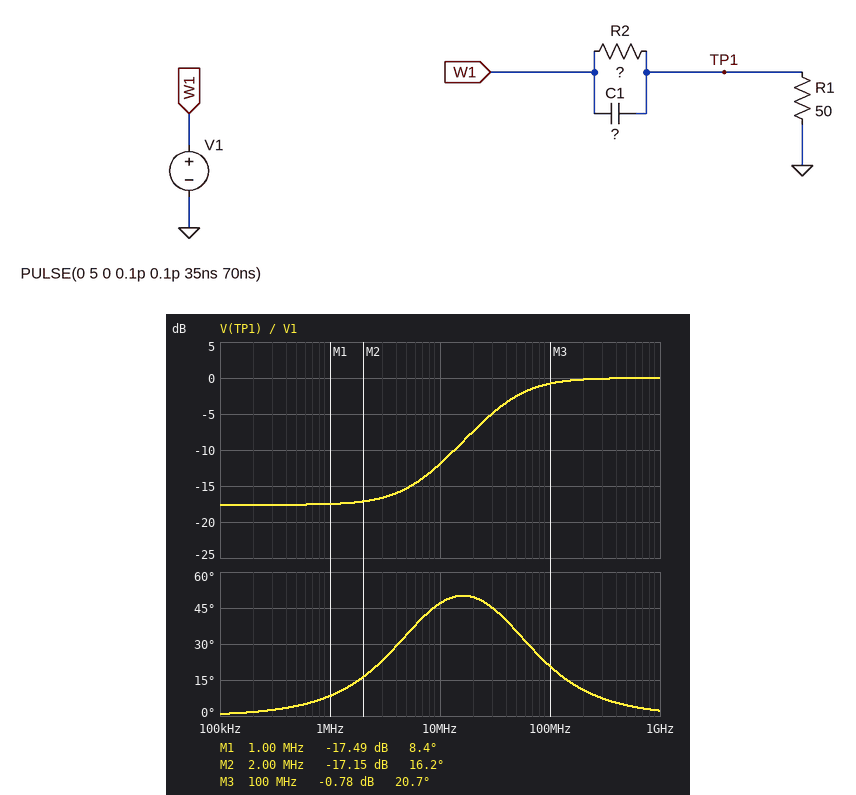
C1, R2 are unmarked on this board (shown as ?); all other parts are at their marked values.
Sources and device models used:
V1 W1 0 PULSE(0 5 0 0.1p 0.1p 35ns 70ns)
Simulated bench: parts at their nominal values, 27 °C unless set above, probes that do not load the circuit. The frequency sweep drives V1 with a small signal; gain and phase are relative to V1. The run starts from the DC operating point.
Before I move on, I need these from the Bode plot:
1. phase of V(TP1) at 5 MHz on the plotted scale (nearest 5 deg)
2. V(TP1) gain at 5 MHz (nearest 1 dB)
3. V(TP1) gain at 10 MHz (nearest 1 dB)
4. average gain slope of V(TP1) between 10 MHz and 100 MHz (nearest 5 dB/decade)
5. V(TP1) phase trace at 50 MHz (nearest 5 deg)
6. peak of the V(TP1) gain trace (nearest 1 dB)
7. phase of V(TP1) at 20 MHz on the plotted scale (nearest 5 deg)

35 deg
-15 dB
-12 dB
10 dB/decade
35 deg
0 dB
50 deg
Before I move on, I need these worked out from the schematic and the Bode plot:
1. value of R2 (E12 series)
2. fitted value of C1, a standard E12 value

330 Ω
82 pF
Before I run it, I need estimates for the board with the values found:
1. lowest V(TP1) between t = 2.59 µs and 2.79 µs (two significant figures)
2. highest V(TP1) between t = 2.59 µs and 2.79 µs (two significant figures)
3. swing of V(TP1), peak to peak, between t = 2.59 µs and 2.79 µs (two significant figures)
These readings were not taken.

-4.3 V
5.0 V
9.3 V
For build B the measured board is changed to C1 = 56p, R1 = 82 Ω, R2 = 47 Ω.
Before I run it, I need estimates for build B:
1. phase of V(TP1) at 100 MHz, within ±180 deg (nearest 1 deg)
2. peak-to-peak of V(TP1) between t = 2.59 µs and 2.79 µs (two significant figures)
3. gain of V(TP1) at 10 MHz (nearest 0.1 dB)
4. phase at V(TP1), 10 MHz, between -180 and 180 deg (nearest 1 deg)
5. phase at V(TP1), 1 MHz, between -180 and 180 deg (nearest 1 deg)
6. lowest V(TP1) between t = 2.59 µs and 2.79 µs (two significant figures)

12 deg
6.8 V
-3.9 dB
3 deg
0 deg
-1.8 V
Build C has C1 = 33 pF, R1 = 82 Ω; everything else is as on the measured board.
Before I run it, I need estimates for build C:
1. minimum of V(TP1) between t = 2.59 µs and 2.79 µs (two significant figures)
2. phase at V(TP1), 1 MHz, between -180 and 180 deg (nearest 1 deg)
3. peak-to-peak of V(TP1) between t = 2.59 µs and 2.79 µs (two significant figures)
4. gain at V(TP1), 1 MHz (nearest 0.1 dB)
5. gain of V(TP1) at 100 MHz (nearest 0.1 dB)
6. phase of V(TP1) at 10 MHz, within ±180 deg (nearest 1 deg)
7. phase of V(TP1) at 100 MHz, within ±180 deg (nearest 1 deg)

-4.0 V
3 deg
9.0 V
-14.0 dB
-1.8 dB
27 deg
28 deg
